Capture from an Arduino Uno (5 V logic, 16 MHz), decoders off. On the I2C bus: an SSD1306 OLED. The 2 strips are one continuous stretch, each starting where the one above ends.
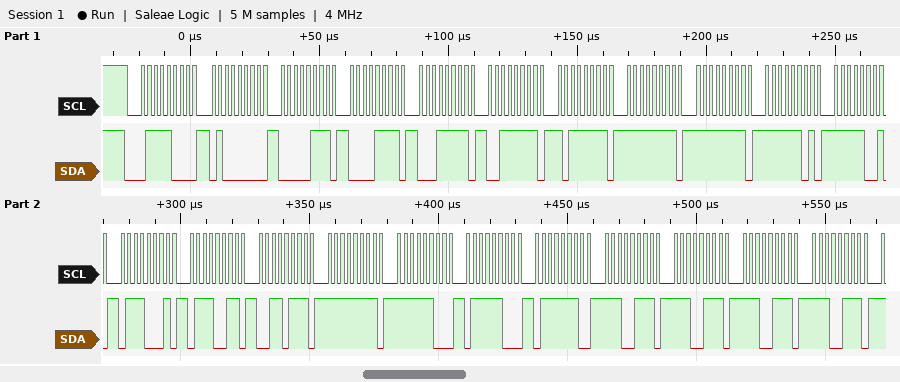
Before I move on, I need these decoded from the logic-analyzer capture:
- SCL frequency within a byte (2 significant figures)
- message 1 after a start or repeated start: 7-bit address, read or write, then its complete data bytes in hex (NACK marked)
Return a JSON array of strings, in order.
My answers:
["400 kHz", "0x3C write: 40 07 0F 1F 3F BF FF FF FD F9 71 73 37 FF FC 7C 7E E7 E7 E7 E7"]
